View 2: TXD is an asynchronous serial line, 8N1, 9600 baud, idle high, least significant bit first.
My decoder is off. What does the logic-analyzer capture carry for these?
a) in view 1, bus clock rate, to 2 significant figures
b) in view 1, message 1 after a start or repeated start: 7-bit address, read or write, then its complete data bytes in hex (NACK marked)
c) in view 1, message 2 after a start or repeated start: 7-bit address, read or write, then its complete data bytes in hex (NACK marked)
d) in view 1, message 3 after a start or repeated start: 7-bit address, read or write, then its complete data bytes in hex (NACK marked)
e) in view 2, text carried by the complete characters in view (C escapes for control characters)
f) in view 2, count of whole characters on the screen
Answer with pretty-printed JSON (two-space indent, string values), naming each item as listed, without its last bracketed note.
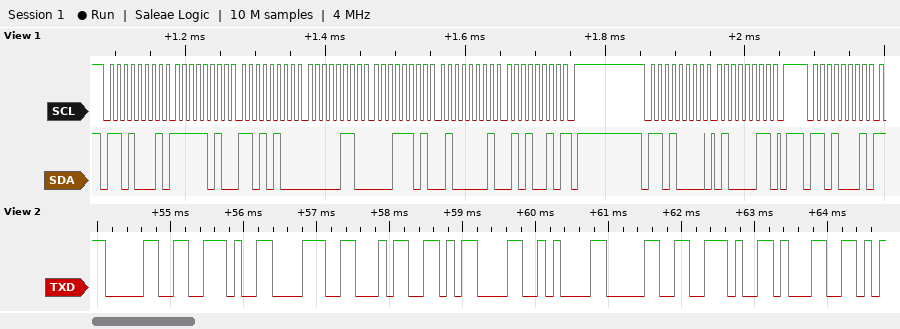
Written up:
{
  "in view 1, bus clock rate, to 2 significant figures": "100 kHz",
  "in view 1, message 1 after a start or repeated start: 7-bit address, read or write, then its complete data bytes in hex": "0x68 read: FA D4 06 1D 41 52 NACK",
  "in view 1, message 2 after a start or repeated start: 7-bit address, read or write, then its complete data bytes in hex": "0x68 write: 43",
  "in view 1, message 3 after a start or repeated start: 7-bit address, read or write, then its complete data bytes in hex": "0x68 read",
  "in view 2, text carried by the complete characters in view": "\"0.84\\r\\n0.1\"",
  "in view 2, count of whole characters on the screen": "9"
}
